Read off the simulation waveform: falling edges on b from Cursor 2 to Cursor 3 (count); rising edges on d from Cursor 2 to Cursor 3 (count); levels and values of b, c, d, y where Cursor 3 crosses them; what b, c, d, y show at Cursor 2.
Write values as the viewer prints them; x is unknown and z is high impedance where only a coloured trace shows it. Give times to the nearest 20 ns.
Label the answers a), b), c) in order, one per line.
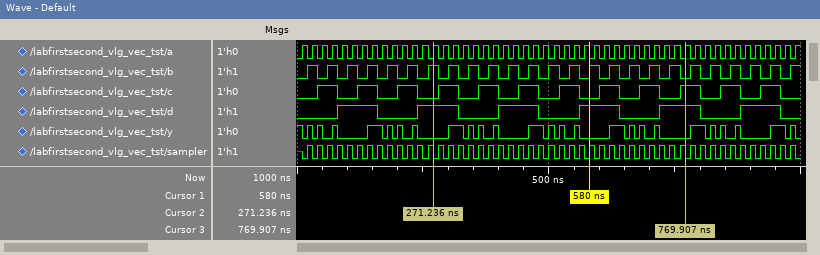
a) 13
b) 3
c) b=0, c=1, d=1, y=0
d) b=1, c=0, d=1, y=0
